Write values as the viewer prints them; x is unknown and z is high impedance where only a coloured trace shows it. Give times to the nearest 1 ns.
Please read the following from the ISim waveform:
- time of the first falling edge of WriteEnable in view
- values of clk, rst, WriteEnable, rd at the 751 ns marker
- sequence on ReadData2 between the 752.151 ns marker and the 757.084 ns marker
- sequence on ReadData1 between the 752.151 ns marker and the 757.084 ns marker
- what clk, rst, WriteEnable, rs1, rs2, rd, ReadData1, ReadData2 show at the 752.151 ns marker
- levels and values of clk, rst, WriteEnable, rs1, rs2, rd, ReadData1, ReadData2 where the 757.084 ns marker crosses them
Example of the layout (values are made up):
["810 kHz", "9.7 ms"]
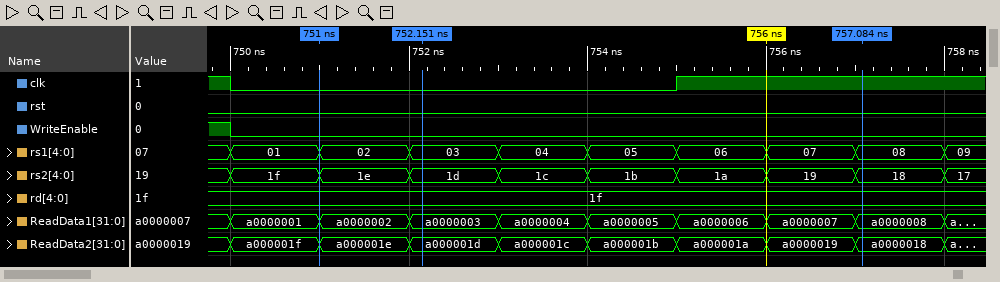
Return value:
["750 ns", "clk=0, rst=0, WriteEnable=0, rd=1f", "a000001d, a000001c, a000001b, a000001a, a0000019, a0000018", "a0000003, a0000004, a0000005, a0000006, a0000007, a0000008", "clk=0, rst=0, WriteEnable=0, rs1=03, rs2=1d, rd=1f, ReadData1=a0000003, ReadData2=a000001d", "clk=1, rst=0, WriteEnable=0, rs1=08, rs2=18, rd=1f, ReadData1=a0000008, ReadData2=a0000018"]
